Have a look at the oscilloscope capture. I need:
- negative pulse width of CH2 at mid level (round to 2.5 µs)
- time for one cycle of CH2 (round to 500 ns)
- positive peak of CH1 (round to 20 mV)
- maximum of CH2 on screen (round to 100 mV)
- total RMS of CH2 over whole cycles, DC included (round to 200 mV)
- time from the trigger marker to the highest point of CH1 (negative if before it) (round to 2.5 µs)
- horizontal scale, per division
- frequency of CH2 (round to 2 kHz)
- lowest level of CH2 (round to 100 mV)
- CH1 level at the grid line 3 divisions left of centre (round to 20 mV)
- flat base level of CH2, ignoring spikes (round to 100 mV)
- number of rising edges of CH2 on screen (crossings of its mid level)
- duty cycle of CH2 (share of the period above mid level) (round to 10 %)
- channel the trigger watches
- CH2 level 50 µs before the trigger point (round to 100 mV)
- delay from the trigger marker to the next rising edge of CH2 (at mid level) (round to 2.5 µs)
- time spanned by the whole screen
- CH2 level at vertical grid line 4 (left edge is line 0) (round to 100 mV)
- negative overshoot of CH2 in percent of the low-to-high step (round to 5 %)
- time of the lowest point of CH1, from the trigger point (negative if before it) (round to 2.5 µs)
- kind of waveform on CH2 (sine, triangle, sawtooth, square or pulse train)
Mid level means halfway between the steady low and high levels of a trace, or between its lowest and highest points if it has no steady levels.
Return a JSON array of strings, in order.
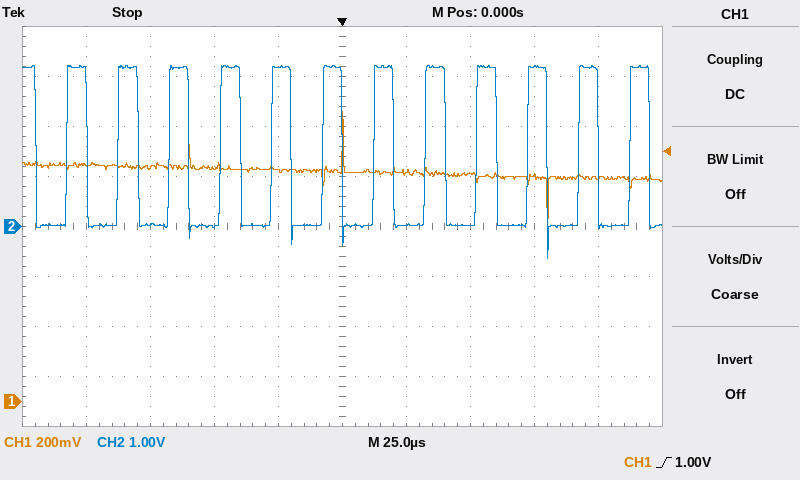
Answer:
["12.5 µs", "20.0 µs", "1.16 V", "3.2 V", "2.0 V", "0.0 µs", "25 µs", "50 kHz", "-600 mV", "940 mV", "0.0 V", "12", "40 %", "CH1", "0.0 V", "12.5 µs", "250 µs", "3.2 V", "20 %", "+80.0 µs", "pulse train"]
